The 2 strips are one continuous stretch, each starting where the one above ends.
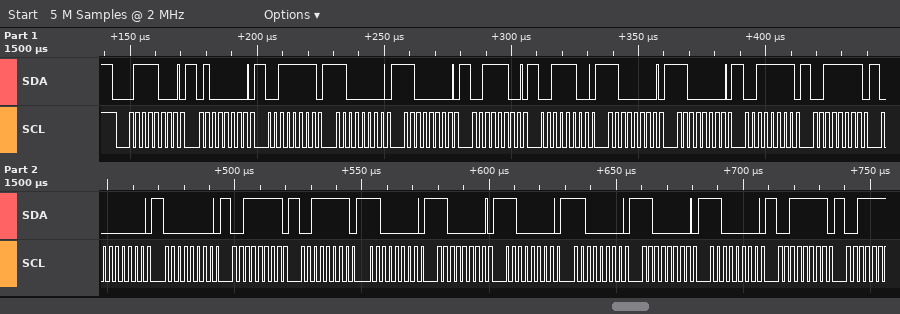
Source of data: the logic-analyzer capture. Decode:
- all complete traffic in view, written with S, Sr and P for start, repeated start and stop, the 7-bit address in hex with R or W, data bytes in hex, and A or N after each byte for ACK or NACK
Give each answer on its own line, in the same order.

S 3CW A 40 A 3F A C0 A C0 A 3C A 3C A C0 A C0 A 3F A 3F A 00 A 00 A 3F A 3F A C0 A C0 A C0 A C0 A C0 A C0 A 3F A
